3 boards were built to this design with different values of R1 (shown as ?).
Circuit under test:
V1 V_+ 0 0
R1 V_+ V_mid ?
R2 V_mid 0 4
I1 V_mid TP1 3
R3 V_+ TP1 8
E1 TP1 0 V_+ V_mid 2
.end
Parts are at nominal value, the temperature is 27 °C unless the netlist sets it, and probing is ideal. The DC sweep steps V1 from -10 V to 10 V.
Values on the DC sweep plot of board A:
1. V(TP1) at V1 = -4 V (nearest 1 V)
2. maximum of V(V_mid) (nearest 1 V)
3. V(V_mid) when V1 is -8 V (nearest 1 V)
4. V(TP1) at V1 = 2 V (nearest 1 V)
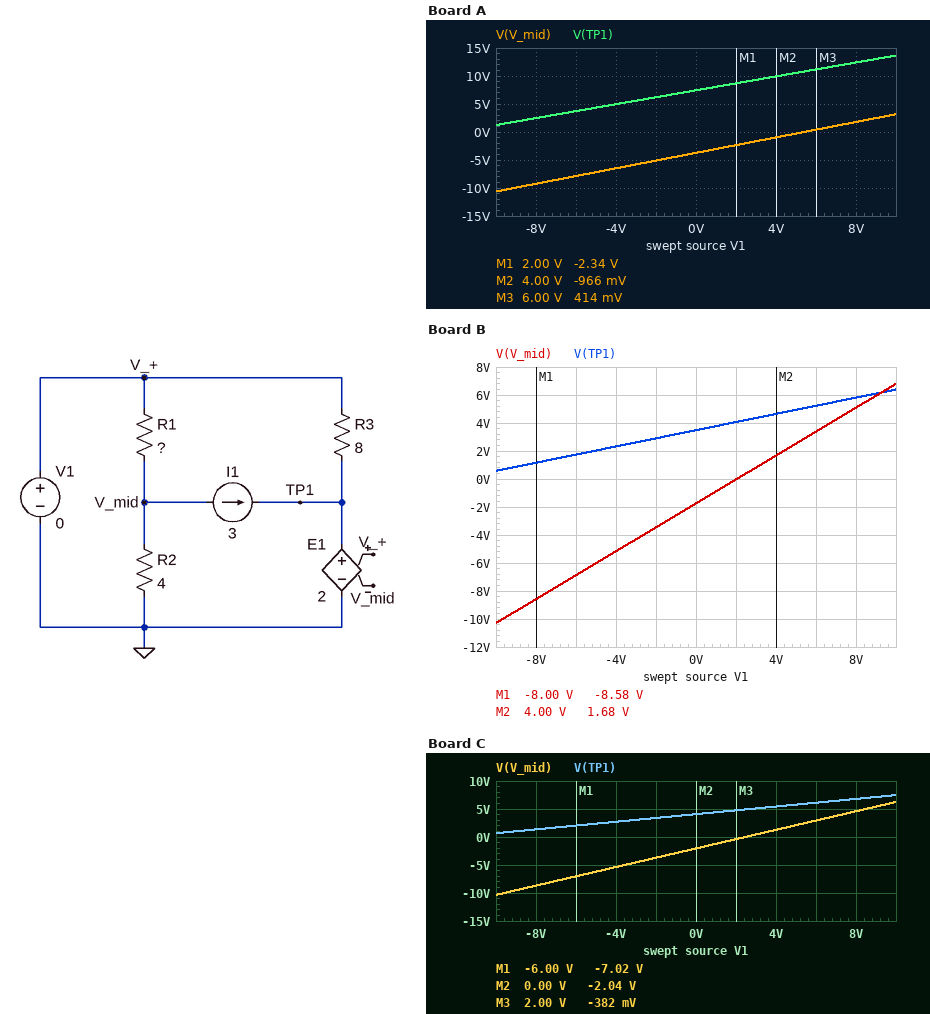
5 V
3 V
-9 V
9 V
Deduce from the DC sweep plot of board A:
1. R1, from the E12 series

1.8 Ω
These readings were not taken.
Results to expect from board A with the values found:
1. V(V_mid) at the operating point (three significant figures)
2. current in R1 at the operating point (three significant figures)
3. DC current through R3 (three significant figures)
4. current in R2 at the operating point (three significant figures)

-3.72 V
2.07 A
931 mA
931 mA
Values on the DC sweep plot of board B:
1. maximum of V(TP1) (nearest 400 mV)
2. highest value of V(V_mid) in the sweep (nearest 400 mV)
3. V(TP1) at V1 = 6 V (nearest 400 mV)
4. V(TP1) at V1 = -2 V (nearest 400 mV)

6.4 V
6.8 V
5.2 V
2.8 V
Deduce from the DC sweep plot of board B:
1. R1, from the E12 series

0.68 Ω
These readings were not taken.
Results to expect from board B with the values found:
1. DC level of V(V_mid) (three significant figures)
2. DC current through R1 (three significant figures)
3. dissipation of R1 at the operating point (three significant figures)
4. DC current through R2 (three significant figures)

-1.74 V
2.56 A
4.47 W
436 mA
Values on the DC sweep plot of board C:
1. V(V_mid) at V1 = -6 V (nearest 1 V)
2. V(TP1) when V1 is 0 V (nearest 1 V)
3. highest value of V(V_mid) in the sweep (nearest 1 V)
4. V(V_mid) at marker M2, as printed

-7 V
4 V
6 V
-2.04 V
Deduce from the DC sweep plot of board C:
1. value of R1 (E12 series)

0.82 Ω
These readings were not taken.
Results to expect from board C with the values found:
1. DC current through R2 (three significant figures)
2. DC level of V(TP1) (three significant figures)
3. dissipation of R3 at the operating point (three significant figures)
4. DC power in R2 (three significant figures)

510 mA
4.08 V
2.08 W
1.04 W
